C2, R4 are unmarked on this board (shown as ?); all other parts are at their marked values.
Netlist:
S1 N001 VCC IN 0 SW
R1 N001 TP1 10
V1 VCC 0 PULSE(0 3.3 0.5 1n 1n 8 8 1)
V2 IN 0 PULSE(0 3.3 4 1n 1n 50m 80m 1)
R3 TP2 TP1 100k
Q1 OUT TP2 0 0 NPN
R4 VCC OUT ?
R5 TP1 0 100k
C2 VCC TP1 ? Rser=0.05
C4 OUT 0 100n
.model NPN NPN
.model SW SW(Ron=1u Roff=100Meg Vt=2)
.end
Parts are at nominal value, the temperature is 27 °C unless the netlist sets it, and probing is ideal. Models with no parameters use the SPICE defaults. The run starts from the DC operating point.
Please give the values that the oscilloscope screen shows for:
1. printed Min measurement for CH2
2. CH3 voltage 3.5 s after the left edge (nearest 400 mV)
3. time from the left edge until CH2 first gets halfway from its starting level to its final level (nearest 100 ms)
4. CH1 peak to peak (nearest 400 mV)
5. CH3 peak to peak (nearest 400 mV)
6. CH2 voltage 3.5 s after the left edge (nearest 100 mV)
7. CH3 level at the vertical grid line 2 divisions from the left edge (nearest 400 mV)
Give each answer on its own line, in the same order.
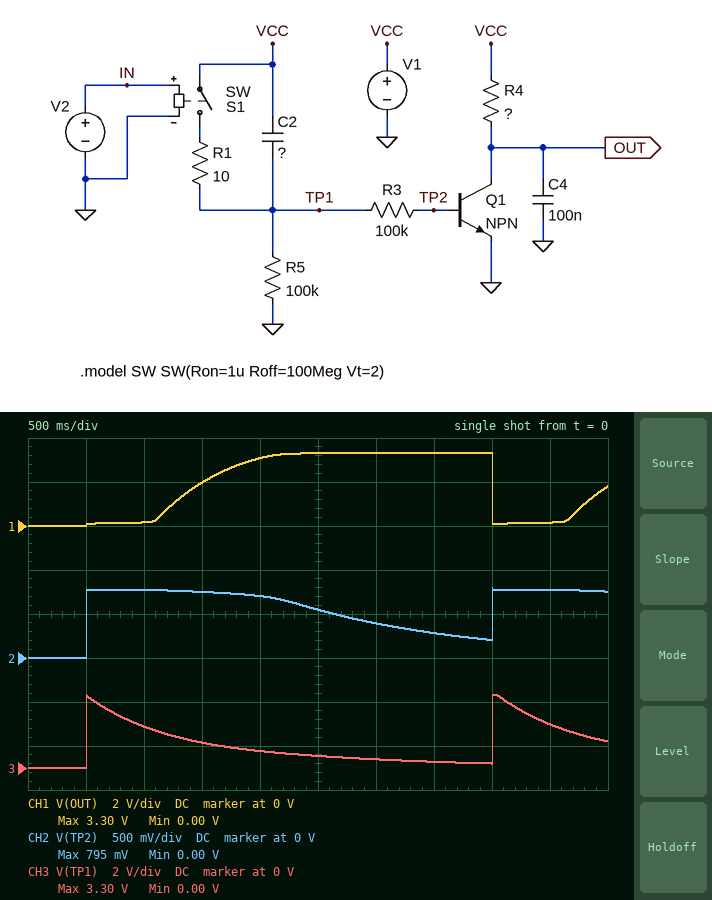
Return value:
0.00 V
400 mV
500 ms
3.2 V
3.2 V
300 mV
2.0 V
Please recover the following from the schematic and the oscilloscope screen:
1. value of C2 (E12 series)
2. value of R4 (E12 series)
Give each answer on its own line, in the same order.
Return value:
15 µF
3.3 kΩ
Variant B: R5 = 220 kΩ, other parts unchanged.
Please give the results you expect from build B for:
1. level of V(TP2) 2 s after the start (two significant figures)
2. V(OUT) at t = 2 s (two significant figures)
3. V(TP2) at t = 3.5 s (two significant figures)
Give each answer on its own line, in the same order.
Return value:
750 mV
1.9 V
640 mV
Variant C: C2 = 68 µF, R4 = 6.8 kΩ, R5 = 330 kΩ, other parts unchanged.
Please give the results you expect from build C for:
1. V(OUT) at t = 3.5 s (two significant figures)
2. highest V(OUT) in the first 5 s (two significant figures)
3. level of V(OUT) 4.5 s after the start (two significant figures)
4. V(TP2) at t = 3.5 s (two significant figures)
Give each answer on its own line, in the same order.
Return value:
100 mV
110 mV
86 mV
760 mV
